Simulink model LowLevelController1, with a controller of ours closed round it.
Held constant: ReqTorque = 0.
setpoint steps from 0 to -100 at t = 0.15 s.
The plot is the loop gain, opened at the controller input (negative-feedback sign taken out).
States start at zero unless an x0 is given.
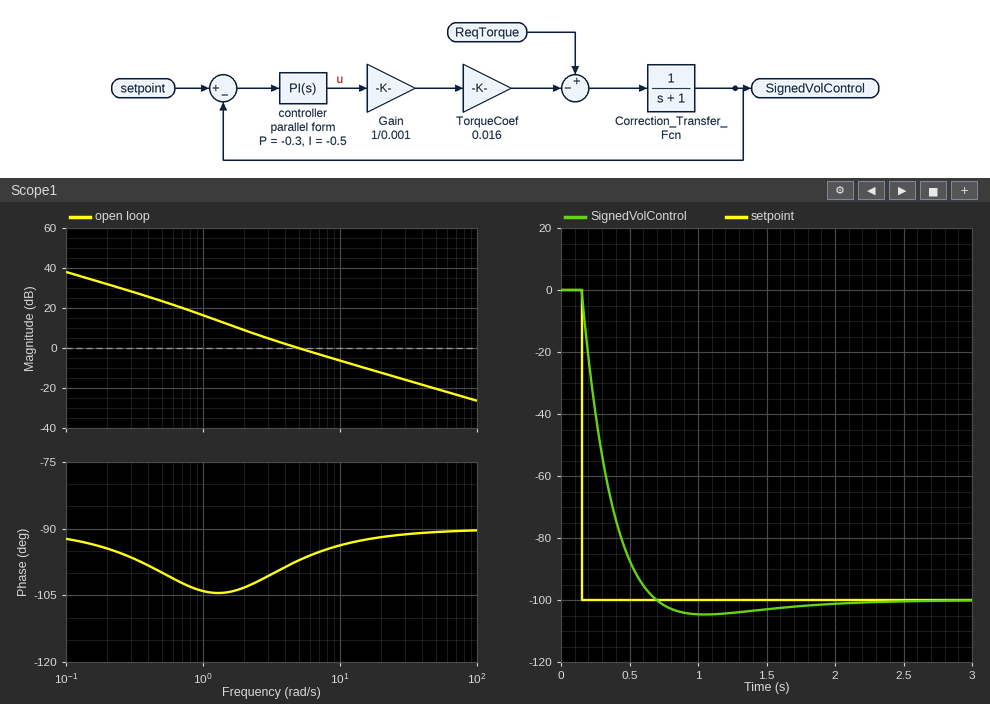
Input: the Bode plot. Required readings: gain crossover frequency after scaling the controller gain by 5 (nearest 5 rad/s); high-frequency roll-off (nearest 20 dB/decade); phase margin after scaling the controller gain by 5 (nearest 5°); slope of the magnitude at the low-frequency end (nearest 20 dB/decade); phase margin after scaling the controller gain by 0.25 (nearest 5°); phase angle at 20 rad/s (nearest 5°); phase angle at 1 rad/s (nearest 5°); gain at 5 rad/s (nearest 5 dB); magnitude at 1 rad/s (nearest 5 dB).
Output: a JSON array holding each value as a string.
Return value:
["25 rad/s", "-20 dB/decade", "90°", "-20 dB/decade", "75°", "-90°", "-105°", "0 dB", "15 dB"]
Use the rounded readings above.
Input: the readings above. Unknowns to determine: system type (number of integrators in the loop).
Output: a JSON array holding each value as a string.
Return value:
["1"]
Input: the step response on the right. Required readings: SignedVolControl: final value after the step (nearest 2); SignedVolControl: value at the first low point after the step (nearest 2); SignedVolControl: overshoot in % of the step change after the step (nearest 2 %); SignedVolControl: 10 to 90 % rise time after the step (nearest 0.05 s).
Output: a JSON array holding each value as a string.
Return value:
["-100", "-104", "4 %", "0.35 s"]
